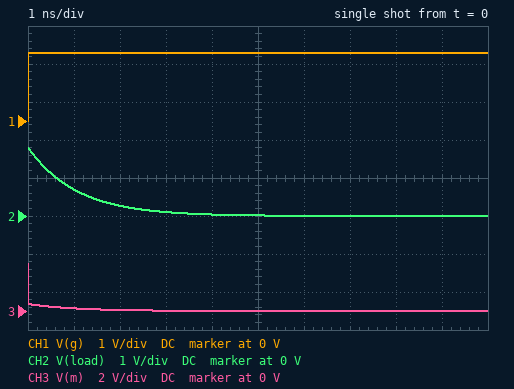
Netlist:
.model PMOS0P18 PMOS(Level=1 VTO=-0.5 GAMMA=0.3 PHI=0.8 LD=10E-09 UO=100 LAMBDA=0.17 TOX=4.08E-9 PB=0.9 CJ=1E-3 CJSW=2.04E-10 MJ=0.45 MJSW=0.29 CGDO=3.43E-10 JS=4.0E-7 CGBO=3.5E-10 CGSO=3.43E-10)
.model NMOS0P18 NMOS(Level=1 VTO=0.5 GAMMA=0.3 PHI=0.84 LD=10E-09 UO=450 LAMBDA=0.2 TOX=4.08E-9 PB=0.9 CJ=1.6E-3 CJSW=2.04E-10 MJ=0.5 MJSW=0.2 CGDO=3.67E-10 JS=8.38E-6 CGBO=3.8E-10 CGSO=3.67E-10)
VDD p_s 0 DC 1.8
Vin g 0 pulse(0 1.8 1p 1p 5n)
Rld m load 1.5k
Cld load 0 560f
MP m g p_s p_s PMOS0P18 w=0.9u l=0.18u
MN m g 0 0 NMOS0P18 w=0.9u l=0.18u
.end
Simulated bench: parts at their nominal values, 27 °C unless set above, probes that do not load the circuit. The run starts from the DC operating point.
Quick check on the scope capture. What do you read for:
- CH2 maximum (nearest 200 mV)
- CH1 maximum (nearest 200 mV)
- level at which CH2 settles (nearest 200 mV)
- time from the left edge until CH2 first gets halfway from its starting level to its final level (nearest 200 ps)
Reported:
1.8 V
1.8 V
0 V
800 ps
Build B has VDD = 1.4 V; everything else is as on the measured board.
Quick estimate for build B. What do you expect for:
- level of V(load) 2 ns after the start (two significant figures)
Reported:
210 mV
